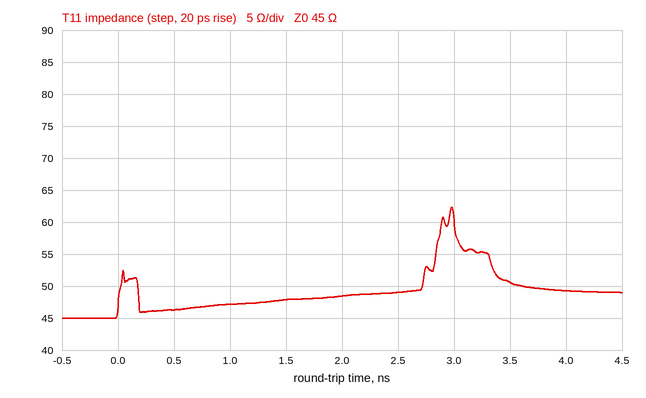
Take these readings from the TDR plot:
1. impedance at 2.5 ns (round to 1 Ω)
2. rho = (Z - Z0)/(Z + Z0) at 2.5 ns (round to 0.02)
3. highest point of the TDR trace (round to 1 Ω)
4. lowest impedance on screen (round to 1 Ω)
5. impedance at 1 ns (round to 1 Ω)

49 Ω
+0.04
62 Ω
45 Ω
47 Ω
